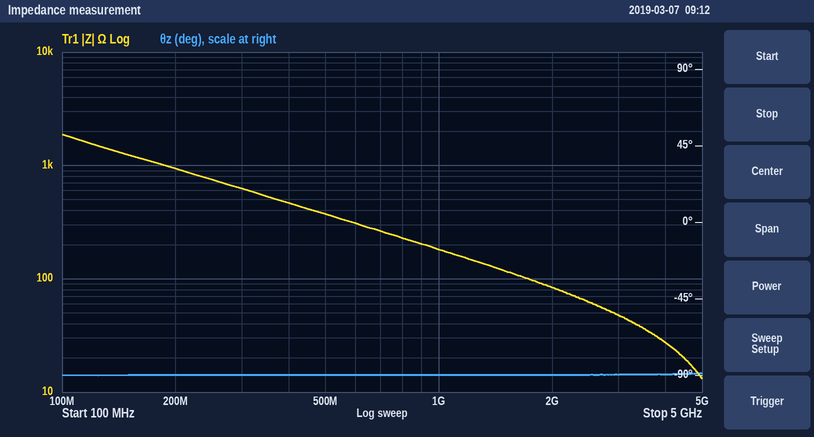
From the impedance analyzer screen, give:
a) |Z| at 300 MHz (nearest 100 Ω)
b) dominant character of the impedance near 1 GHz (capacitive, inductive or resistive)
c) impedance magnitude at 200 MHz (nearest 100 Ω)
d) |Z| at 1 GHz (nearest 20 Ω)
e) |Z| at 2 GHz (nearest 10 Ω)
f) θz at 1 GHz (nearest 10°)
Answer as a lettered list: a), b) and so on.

a) 600 Ω
b) capacitive
c) 900 Ω
d) 180 Ω
e) 80 Ω
f) -90°
